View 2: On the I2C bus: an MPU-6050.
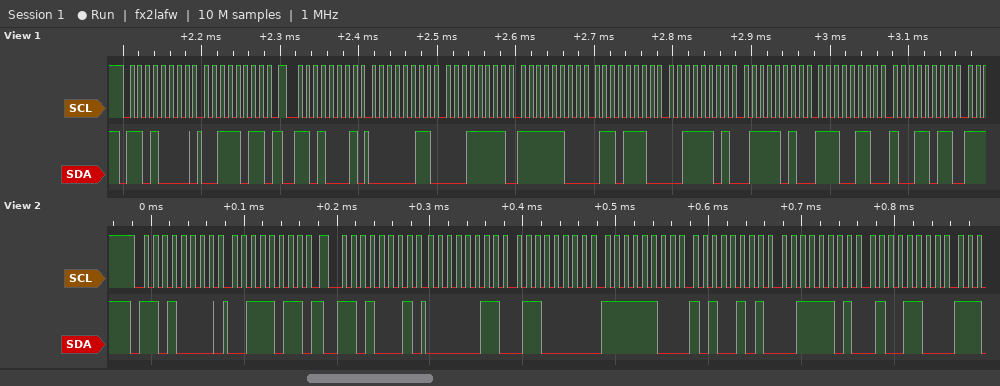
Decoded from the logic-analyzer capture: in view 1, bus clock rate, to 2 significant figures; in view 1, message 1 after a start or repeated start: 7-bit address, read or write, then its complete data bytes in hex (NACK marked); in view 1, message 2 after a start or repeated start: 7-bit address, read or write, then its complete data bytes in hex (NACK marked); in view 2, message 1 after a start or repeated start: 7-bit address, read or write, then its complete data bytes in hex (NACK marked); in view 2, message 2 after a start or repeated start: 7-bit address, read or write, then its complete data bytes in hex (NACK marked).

100 kHz
0x68 write: 3B
0x68 read: 03 1F FC 6E 3D 7A E6 9B
0x68 write: 3B
0x68 read: 03 60 FC A5 3D 4C
